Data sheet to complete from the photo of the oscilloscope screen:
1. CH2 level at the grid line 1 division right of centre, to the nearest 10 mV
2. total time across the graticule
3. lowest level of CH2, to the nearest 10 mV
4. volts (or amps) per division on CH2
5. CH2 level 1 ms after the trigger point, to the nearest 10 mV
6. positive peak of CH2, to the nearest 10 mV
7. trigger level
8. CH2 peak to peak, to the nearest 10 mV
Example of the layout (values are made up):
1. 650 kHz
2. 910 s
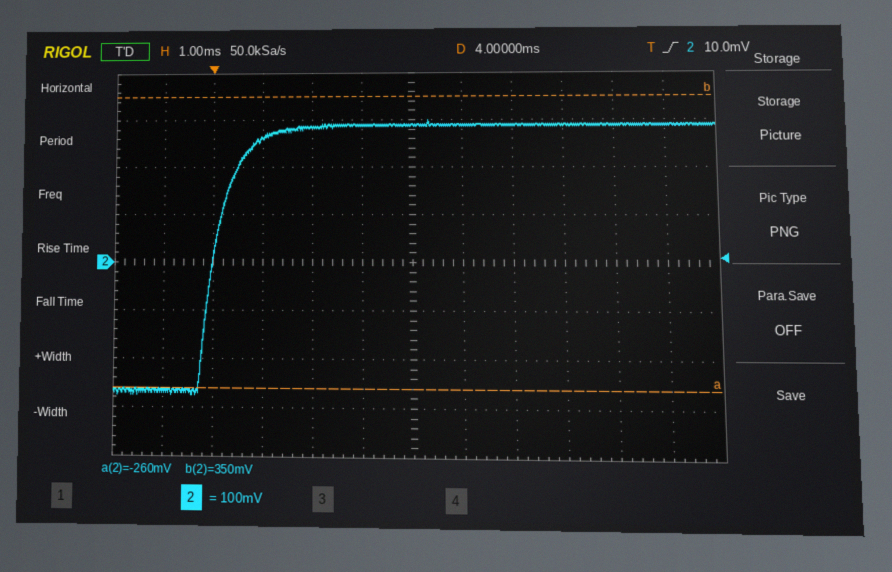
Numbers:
1. 290 mV
2. 12 ms
3. -270 mV
4. 100 mV
5. 260 mV
6. 300 mV
7. 10.0 mV
8. 570 mV
